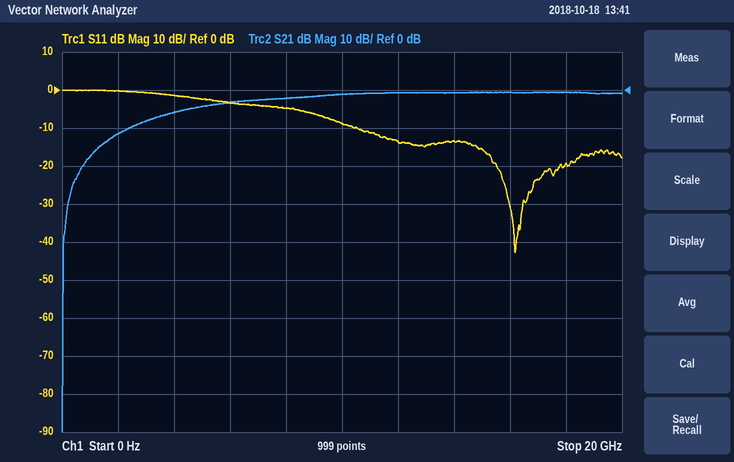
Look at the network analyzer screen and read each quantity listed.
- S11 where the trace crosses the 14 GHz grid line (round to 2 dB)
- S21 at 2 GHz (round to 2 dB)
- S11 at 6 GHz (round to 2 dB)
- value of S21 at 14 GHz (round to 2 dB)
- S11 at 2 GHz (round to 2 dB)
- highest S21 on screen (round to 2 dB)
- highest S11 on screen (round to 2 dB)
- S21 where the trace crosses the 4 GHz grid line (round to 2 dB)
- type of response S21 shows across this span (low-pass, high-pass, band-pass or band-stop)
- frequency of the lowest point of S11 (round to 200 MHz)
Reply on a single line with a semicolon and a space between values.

-14 dB; -12 dB; -4 dB; 0 dB; 0 dB; 0 dB; 0 dB; -6 dB; high-pass; 16.2 GHz
